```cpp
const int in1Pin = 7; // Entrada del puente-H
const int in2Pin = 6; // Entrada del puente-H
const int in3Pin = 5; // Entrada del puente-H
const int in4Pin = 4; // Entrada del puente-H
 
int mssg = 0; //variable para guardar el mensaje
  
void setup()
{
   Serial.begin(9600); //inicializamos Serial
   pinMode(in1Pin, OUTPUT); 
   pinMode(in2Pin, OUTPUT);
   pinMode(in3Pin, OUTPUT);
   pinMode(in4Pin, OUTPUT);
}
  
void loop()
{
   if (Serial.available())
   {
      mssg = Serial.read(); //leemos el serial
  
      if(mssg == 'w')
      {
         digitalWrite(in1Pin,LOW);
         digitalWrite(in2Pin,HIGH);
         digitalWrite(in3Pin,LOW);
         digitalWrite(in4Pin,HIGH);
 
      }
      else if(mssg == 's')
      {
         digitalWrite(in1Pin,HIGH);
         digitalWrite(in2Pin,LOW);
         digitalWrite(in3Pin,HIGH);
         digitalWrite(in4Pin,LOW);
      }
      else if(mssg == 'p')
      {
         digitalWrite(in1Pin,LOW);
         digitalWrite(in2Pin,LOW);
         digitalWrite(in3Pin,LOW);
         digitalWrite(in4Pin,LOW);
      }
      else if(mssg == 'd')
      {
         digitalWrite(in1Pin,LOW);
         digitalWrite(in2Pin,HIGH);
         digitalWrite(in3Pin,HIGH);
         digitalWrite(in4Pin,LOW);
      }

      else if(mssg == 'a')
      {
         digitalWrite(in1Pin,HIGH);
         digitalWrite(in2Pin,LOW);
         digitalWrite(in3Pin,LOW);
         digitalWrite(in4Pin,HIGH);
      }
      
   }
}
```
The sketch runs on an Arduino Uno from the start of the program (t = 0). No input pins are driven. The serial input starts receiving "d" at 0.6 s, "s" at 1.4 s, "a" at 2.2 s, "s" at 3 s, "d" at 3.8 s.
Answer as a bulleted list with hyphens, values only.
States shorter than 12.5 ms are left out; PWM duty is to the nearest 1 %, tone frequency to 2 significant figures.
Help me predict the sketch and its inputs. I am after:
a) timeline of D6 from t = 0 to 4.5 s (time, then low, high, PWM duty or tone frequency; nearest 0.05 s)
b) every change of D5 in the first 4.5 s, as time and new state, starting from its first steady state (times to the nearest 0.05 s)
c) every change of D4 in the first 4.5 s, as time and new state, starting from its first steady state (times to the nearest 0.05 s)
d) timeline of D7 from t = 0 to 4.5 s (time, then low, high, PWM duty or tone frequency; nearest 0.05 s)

- 0 s low; 0.6 s high; 1.4 s low; 3.8 s high
- 0 s low; 0.6 s high; 2.2 s low; 3 s high
- 0 s low; 2.2 s high; 3 s low
- 0 s low; 1.4 s high; 3.8 s low
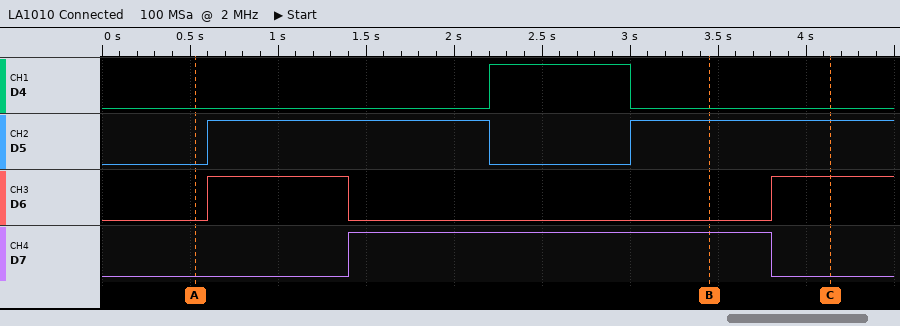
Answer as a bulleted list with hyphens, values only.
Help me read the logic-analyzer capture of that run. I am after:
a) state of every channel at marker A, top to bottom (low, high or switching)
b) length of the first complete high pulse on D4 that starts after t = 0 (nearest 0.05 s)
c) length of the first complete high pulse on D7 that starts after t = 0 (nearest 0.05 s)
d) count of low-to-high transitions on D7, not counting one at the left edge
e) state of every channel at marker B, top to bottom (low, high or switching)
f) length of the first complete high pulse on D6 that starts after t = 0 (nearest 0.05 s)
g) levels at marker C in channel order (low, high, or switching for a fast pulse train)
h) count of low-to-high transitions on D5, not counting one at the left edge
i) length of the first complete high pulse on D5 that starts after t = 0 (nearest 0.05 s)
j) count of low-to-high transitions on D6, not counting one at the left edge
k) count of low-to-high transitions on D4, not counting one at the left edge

- D4 low, D5 low, D6 low, D7 low
- 0.80 s
- 2.40 s
- 1
- D4 low, D5 high, D6 low, D7 high
- 0.80 s
- D4 low, D5 high, D6 high, D7 low
- 2
- 1.60 s
- 2
- 1
